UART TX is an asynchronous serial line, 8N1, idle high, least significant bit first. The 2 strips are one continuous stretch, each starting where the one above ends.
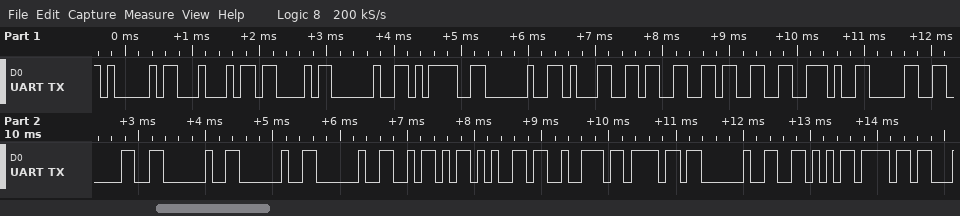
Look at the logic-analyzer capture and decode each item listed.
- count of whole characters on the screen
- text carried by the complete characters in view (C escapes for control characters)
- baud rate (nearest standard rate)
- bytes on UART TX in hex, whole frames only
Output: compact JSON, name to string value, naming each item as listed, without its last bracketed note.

{"count of whole characters on the screen": "22", "text carried by the complete characters in view": "\"ADC = 133.00   Zero Vo\"", "baud rate": "9600 baud", "bytes on UART TX in hex, whole frames only": "41 44 43 20 3D 20 31 33 33 2E 30 30 20 20 20 5A 65 72 6F 20 56 6F"}
